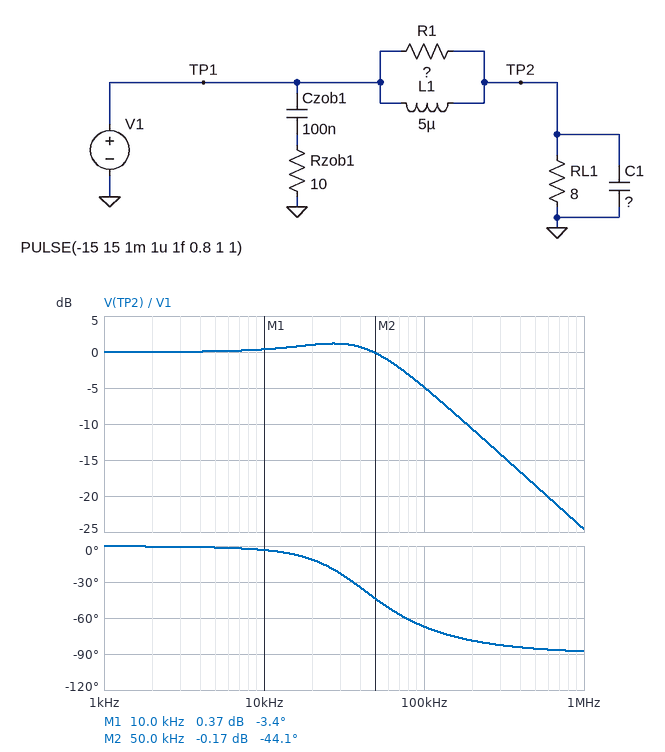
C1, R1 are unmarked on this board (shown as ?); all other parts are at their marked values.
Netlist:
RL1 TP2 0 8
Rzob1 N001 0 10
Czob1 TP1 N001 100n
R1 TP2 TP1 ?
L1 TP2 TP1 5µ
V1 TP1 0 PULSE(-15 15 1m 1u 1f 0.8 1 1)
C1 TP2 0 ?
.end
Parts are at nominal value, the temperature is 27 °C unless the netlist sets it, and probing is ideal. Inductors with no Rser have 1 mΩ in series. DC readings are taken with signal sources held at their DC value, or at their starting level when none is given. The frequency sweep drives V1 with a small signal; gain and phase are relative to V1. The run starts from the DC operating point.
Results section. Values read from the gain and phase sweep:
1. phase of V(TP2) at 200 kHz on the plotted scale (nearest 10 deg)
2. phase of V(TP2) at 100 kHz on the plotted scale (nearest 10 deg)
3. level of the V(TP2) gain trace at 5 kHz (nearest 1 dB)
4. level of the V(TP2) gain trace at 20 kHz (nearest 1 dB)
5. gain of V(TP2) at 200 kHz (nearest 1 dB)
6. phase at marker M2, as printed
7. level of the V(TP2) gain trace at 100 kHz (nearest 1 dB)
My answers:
-80 deg
-70 deg
0 dB
1 dB
-11 dB
-44.1 deg
-5 dB
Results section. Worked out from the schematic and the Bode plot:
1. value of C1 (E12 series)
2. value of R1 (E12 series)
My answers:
3.3 µF
0.82 Ω
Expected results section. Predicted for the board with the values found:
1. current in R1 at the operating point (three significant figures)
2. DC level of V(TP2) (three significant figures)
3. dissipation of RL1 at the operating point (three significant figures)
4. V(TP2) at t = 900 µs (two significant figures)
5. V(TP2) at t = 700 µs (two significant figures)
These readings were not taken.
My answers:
2.28 mA
-15.0 V
28.1 W
-15 V
-15 V
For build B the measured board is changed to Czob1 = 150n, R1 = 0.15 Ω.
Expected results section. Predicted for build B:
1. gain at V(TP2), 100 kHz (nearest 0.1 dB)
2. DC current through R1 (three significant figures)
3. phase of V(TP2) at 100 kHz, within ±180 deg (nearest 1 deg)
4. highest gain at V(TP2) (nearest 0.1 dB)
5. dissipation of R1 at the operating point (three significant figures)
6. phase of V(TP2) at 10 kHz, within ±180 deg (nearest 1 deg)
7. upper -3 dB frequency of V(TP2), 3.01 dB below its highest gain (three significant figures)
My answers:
-0.4 dB
12.4 mA
-17 deg
0 dB
23.1 µW
-2 deg
320 kHz
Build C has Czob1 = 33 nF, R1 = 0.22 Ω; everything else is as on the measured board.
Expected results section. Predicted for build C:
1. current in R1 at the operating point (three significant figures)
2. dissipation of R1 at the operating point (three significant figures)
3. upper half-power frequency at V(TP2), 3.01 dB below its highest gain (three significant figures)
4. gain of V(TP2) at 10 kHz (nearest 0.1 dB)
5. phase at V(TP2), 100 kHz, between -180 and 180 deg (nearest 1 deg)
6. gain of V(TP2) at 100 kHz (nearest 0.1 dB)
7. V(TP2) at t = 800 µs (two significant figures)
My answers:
8.48 mA
15.8 µW
219 kHz
0 dB
-25 deg
-0.8 dB
-15 V
